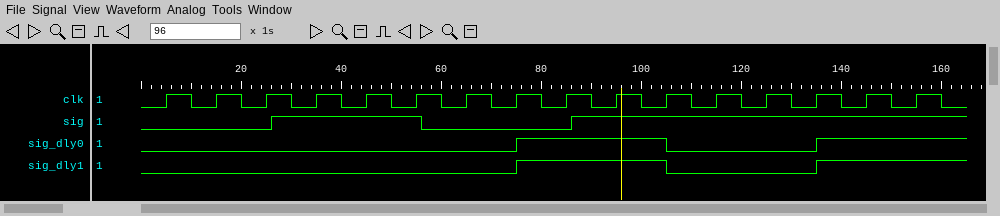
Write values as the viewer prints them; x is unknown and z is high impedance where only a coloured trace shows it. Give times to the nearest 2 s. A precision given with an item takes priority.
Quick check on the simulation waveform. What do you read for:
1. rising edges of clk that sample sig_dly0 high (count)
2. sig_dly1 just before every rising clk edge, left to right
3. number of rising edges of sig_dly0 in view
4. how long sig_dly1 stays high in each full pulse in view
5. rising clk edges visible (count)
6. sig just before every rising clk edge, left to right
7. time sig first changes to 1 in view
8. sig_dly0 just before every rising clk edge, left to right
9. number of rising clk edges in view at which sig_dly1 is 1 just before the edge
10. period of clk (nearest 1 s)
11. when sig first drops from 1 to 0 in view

5
0 0 0 0 0 0 0 0 1 1 1 0 0 0 1 1
2
30 s
16
0 0 0 1 1 1 0 0 0 1 1 1 1 1 1 1
26 s
0 0 0 0 0 0 0 0 1 1 1 0 0 0 1 1
5
10 s
56 s
